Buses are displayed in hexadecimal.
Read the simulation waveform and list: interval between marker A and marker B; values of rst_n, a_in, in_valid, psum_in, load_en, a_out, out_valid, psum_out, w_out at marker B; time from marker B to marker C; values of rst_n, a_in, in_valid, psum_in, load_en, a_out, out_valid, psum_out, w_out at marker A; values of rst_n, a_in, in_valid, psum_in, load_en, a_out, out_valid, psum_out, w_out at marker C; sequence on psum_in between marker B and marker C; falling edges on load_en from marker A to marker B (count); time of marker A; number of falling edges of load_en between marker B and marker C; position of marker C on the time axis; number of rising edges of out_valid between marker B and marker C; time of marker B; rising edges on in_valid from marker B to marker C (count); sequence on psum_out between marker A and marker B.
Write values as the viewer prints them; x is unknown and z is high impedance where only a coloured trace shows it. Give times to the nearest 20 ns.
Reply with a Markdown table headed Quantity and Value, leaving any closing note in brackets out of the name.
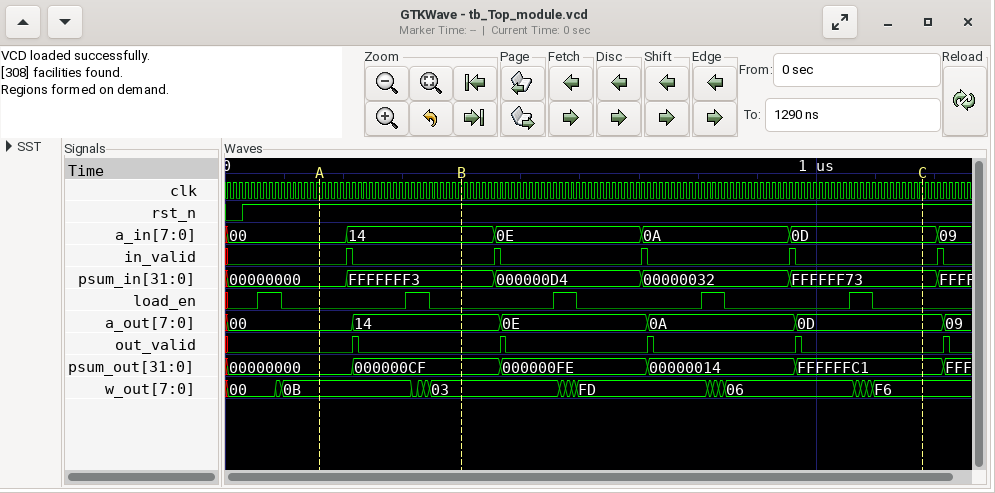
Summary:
| Quantity | Value |
|---|---|
| interval between marker A and marker B | 240 ns |
| values of rst_n, a_in, in_valid, psum_in, load_en, a_out, out_valid, psum_out, w_out at marker B | rst_n=1, a_in=14, in_valid=0, psum_in=FFFFFFF3, load_en=0, a_out=14, out_valid=0, psum_out=000000CF, w_out=03 |
| time from marker B to marker C | 780 ns |
| values of rst_n, a_in, in_valid, psum_in, load_en, a_out, out_valid, psum_out, w_out at marker A | rst_n=1, a_in=00, in_valid=0, psum_in=00000000, load_en=0, a_out=00, out_valid=0, psum_out=00000000, w_out=0B |
| values of rst_n, a_in, in_valid, psum_in, load_en, a_out, out_valid, psum_out, w_out at marker C | rst_n=1, a_in=0D, in_valid=0, psum_in=FFFFFF73, load_en=0, a_out=0D, out_valid=0, psum_out=FFFFFFC1, w_out=F6 |
| sequence on psum_in between marker B and marker C | FFFFFFF3, 000000D4, 00000032, FFFFFF73 |
| falling edges on load_en from marker A to marker B | 1 |
| time of marker A | 160 ns |
| number of falling edges of load_en between marker B and marker C | 3 |
| position of marker C on the time axis | 1180 ns |
| number of rising edges of out_valid between marker B and marker C | 3 |
| time of marker B | 400 ns |
| rising edges on in_valid from marker B to marker C | 3 |
| sequence on psum_out between marker A and marker B | 00000000, 000000CF |
